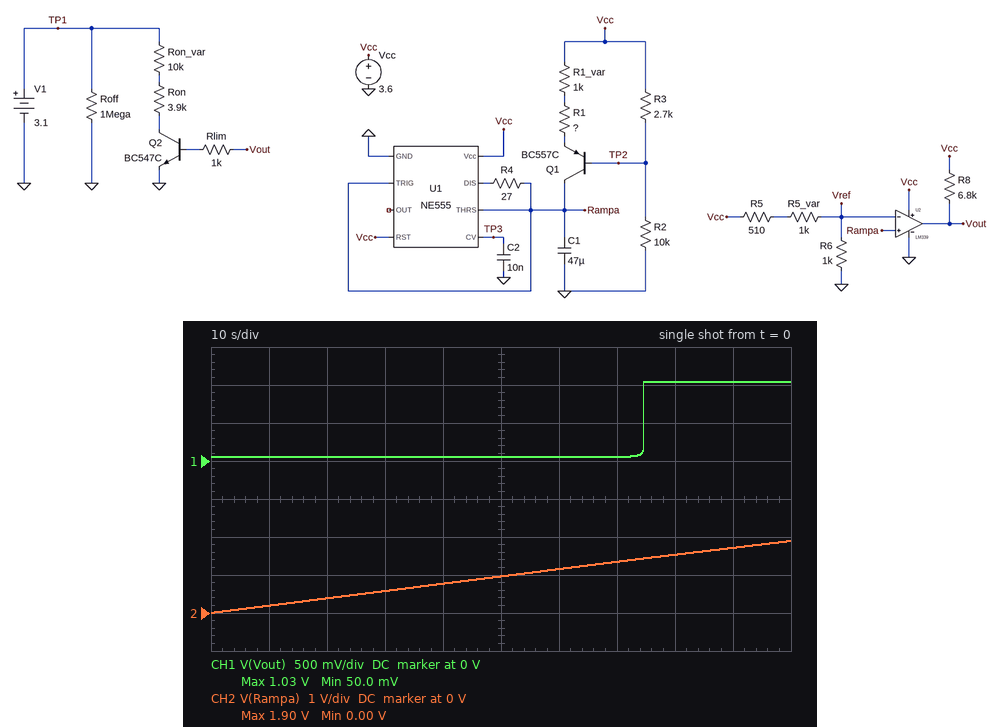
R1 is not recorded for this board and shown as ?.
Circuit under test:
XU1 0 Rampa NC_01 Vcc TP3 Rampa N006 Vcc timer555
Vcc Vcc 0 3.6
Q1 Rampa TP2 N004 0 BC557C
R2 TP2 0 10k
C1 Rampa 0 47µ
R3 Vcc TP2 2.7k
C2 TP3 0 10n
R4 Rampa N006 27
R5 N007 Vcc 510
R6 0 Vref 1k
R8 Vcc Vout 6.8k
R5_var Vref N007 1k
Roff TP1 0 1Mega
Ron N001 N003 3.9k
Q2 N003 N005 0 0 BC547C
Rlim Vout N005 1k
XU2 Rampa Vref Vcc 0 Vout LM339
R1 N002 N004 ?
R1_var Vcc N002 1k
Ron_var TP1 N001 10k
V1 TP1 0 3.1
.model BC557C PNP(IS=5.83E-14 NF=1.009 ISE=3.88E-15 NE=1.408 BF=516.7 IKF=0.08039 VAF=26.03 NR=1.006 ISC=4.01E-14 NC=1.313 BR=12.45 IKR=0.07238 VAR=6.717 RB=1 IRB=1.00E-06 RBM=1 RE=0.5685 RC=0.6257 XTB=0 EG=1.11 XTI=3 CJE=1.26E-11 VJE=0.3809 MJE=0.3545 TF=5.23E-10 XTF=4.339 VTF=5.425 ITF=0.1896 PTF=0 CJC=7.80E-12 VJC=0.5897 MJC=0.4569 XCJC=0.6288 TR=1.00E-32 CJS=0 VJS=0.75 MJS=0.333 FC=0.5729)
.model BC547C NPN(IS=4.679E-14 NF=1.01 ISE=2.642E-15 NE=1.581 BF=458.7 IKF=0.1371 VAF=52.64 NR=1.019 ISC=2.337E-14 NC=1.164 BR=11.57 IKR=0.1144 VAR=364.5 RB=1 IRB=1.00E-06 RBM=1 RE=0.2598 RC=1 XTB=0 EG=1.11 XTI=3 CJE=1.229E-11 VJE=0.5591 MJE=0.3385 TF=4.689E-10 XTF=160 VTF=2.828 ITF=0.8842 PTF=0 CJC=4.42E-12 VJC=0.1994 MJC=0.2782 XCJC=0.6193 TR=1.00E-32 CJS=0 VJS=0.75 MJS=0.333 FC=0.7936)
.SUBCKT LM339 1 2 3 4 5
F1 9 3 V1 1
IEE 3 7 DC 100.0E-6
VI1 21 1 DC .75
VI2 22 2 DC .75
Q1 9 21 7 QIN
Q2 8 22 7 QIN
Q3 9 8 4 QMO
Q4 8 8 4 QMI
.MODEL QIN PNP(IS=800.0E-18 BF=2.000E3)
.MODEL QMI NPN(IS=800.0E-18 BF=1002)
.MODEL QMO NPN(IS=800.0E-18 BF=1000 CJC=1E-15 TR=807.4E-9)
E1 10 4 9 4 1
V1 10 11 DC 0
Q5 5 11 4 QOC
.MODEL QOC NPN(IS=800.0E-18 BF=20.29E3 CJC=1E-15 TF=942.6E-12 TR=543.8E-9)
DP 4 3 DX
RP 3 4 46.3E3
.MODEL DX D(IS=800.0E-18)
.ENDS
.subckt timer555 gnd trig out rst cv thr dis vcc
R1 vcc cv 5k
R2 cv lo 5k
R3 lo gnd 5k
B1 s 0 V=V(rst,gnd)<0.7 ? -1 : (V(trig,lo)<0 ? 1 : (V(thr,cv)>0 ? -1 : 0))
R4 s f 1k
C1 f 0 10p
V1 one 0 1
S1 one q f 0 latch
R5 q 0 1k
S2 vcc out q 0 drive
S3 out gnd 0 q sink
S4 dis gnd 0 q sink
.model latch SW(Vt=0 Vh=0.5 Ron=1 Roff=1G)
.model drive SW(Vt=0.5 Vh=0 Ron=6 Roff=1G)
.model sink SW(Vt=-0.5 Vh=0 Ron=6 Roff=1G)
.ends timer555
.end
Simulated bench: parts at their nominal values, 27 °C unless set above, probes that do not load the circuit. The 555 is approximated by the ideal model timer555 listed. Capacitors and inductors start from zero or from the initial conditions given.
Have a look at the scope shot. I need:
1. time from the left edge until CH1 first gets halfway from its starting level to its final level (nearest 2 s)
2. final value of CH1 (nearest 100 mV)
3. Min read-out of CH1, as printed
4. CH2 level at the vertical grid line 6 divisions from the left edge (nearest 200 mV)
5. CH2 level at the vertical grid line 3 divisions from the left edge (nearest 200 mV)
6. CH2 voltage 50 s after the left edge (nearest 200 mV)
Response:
74 s
1.0 V
50.0 mV
1.2 V
600 mV
1.0 V
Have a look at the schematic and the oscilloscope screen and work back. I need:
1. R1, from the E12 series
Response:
390 kΩ
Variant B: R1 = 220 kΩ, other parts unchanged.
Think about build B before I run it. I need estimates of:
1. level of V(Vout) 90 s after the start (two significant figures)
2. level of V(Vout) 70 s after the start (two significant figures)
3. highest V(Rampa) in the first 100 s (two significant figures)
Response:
1.0 V
1.0 V
2.4 V
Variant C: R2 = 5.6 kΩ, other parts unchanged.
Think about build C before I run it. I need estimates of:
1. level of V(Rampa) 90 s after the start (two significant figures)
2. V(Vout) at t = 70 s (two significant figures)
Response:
2.4 V
1.0 V
